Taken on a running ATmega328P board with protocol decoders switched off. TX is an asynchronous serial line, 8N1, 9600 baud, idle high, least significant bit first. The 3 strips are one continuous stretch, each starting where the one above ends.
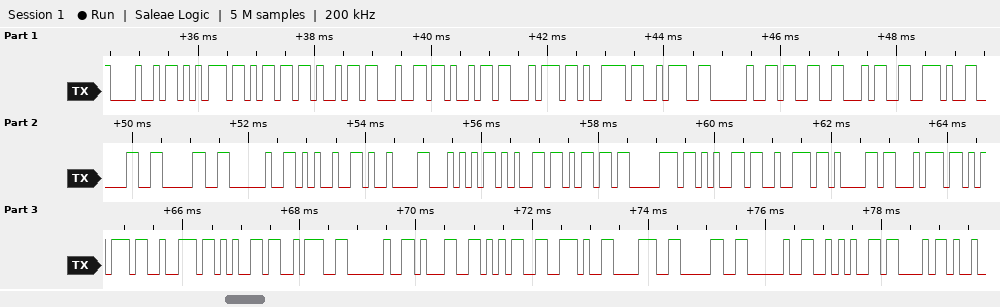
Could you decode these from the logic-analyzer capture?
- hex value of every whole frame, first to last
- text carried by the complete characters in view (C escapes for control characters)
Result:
48 75 6D 69 64 69 74 79 3A 20 33 34 2E 30 30 20 25 09 54 65 6D 70 65 72 61 74 75 72 65 3A 20 31 35 2E 38 30 20 2A 43
"Humidity: 34.00 %\tTemperature: 15.80 *C"
